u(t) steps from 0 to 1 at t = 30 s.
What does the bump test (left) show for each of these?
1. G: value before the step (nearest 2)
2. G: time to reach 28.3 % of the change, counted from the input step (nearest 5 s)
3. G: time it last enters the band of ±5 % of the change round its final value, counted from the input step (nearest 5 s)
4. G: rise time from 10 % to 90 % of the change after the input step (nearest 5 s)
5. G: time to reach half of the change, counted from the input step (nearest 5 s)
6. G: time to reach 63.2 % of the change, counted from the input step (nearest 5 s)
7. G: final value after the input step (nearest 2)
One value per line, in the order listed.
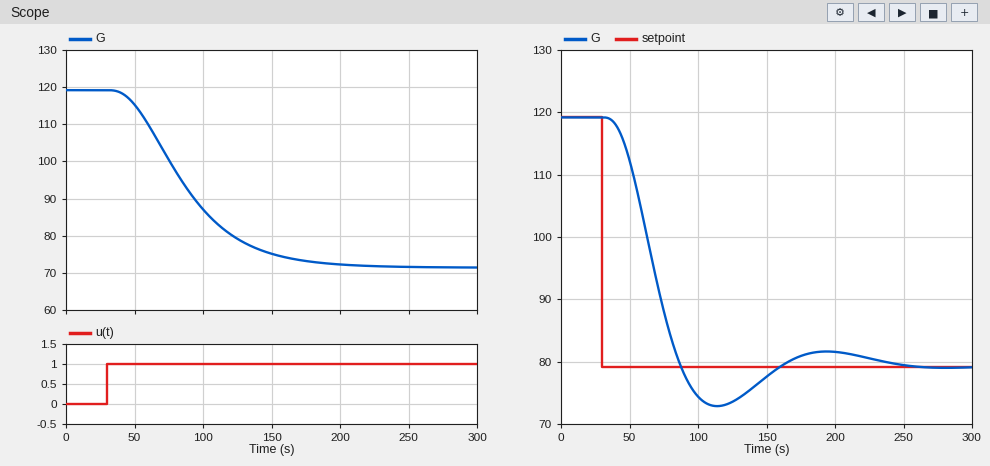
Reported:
120
35 s
135 s
90 s
55 s
65 s
72
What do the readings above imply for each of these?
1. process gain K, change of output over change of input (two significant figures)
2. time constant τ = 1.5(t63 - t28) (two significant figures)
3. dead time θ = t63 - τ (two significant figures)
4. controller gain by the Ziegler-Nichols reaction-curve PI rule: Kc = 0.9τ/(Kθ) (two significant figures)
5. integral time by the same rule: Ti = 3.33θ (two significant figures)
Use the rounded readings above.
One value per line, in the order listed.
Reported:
-48
45 s
20 s
-0.042
67 s
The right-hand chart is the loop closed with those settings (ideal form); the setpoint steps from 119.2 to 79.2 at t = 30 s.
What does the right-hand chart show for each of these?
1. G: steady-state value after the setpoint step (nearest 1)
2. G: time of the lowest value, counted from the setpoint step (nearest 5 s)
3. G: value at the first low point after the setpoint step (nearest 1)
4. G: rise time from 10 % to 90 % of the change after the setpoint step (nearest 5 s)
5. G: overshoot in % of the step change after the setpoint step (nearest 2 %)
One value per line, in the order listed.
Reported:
79
85 s
73
35 s
16 %
